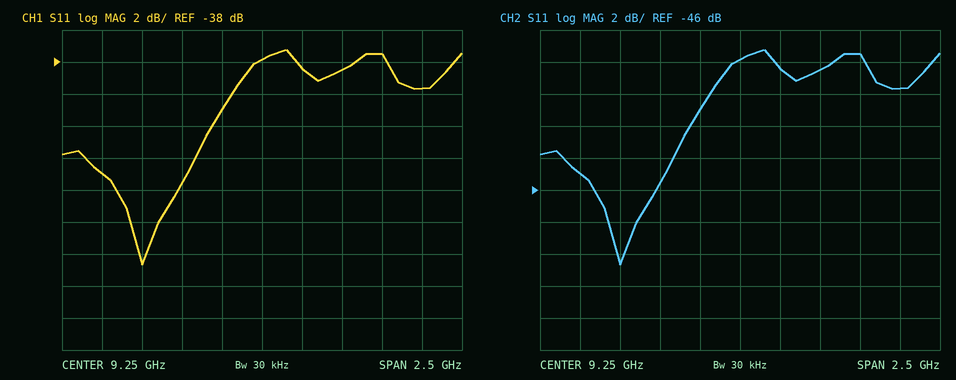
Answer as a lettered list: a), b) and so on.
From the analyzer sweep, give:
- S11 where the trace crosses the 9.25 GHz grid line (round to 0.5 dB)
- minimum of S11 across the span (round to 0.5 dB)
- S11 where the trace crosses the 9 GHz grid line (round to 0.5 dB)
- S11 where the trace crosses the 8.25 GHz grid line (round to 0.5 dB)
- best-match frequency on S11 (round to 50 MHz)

a) -38.0 dB
b) -50.5 dB
c) -41.0 dB
d) -45.0 dB
e) 8.50 GHz
